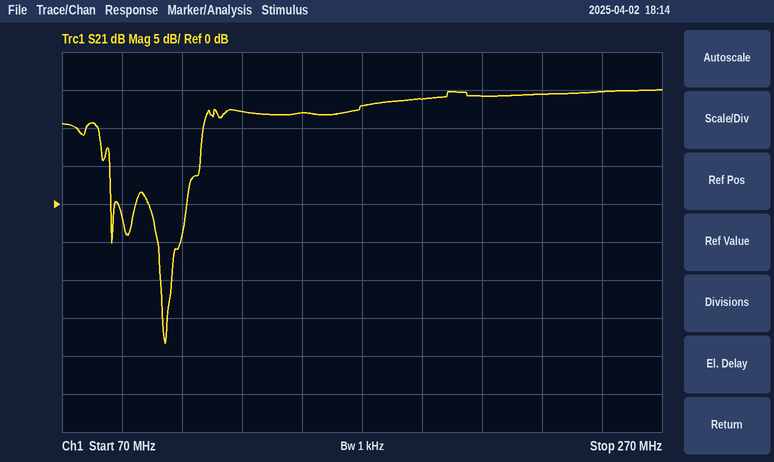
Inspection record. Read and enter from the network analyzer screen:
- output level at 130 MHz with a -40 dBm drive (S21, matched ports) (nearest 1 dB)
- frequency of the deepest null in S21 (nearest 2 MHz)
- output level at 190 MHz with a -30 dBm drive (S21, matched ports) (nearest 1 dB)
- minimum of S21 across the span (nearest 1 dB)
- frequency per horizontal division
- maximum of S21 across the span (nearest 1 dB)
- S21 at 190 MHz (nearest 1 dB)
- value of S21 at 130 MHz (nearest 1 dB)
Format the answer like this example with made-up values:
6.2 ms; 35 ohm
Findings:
-28 dBm; 104 MHz; -16 dBm; -18 dB; 20 MHz; 15 dB; 14 dB; 12 dB
